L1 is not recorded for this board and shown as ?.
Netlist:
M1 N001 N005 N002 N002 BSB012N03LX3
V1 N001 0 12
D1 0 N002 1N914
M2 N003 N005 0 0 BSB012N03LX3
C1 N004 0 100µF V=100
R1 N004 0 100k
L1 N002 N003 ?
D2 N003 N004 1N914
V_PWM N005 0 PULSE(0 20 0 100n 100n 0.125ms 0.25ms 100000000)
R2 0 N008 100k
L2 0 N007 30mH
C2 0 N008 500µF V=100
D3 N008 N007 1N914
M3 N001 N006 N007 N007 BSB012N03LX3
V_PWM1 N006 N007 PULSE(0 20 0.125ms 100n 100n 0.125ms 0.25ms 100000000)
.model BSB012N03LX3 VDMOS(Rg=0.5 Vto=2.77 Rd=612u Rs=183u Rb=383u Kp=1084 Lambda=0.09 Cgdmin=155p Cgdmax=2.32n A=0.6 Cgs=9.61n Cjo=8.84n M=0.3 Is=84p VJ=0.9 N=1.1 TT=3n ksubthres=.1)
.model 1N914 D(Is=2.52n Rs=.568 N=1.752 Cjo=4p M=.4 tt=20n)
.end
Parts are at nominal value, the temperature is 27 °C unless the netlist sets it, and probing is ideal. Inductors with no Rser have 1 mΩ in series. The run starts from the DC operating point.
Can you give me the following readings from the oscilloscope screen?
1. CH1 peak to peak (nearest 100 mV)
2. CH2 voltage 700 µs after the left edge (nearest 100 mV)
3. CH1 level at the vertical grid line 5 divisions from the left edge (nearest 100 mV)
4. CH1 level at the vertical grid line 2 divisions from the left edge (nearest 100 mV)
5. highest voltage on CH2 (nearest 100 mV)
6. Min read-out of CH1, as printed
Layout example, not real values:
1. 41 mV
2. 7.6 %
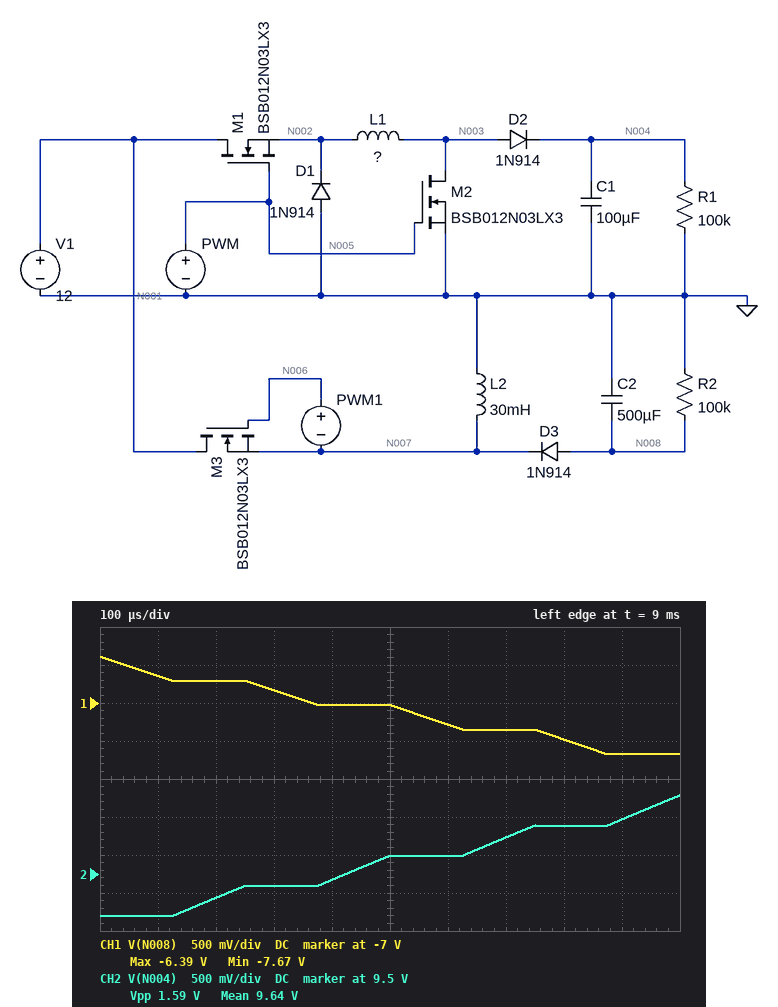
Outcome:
1. 1.3 V
2. 10.0 V
3. -7.0 V
4. -6.7 V
5. 10.5 V
6. -7.67 V
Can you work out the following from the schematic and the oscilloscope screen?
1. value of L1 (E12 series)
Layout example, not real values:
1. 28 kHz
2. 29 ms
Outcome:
1. 100 mH
